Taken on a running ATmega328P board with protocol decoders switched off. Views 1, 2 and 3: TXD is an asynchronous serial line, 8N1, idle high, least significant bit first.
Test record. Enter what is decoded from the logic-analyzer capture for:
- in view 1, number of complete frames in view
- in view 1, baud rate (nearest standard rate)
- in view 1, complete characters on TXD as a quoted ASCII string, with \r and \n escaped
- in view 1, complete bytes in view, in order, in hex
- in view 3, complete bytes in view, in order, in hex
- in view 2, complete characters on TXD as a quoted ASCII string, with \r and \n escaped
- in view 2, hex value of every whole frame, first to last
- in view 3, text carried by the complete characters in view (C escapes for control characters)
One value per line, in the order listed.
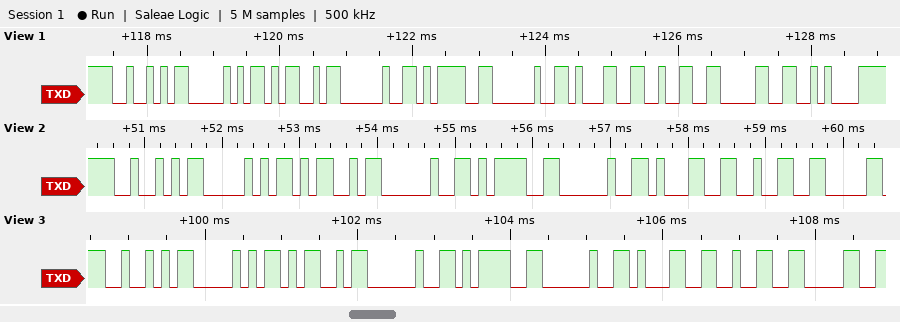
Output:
10
9600 baud
"RPM = 120\n"
52 50 4D 20 3D 20 31 32 30 0A
52 50 4D 20 3D 20 31 32 30
"RPM = 12"
52 50 4D 20 3D 20 31 32
"RPM = 120"
